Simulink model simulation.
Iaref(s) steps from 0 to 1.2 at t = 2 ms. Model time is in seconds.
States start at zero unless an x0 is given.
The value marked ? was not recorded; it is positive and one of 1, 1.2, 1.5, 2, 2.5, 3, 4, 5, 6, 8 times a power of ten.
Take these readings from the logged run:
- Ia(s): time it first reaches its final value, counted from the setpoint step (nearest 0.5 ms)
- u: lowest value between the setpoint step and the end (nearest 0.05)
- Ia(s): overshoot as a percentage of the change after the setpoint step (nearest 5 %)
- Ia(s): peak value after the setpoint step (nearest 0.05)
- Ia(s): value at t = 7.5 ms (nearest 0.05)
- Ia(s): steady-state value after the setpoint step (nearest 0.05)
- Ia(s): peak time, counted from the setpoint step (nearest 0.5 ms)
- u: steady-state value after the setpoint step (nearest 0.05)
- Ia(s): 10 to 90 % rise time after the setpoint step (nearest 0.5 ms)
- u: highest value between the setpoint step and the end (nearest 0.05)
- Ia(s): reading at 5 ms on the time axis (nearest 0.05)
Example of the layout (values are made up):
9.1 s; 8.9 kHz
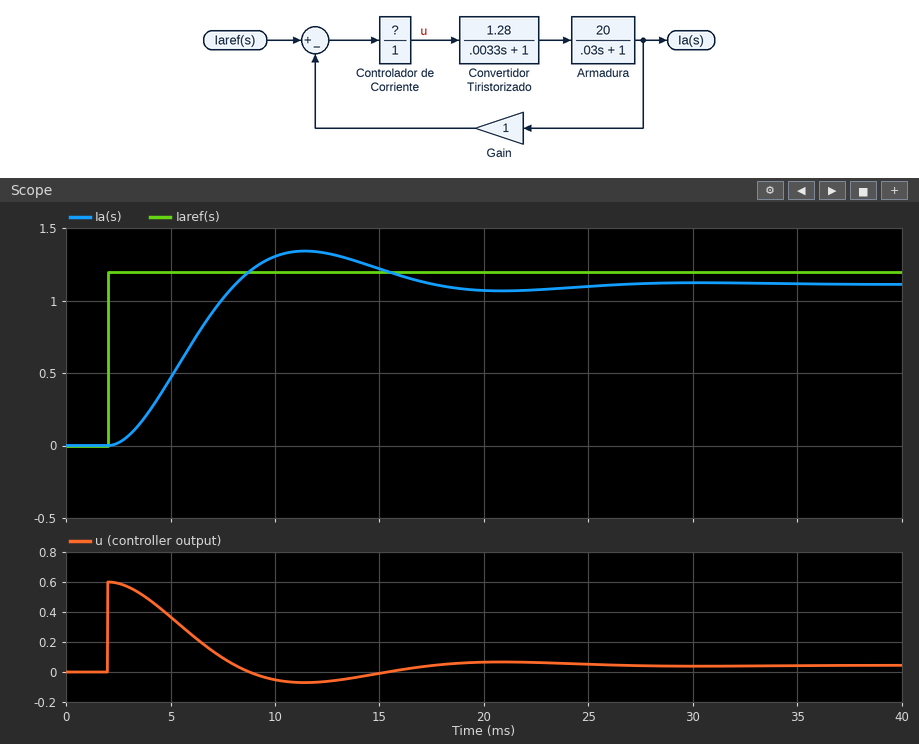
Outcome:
6.0 ms; -0.05; 20 %; 1.35; 1.00; 1.10; 9.5 ms; 0.05; 4.0 ms; 0.60; 0.45
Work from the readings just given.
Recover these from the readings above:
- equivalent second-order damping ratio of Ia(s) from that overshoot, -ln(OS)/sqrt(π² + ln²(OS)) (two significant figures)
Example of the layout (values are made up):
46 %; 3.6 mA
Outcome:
0.46
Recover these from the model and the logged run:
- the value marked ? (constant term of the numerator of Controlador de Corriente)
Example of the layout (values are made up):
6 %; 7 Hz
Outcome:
0.5
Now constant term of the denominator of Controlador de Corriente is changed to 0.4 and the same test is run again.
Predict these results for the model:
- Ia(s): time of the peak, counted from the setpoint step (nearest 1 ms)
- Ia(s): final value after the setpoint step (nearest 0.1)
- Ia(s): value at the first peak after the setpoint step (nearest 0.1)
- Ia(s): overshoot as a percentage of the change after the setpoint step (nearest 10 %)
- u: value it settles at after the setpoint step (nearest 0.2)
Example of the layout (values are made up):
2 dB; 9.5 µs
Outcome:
6 ms; 1.2; 1.6; 40 %; 0.0
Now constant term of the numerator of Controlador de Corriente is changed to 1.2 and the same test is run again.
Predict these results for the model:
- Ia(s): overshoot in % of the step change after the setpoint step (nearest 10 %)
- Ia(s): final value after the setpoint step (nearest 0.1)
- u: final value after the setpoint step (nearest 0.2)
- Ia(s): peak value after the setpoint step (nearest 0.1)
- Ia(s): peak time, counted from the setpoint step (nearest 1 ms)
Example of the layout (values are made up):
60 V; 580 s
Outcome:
40 %; 1.2; 0.0; 1.6; 6 ms
